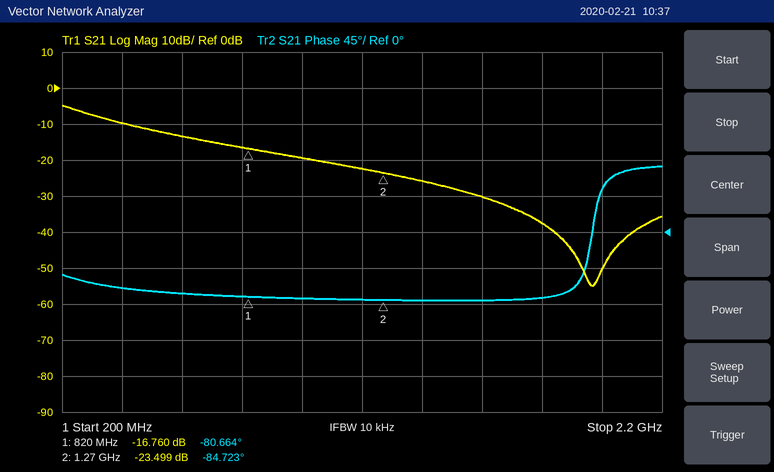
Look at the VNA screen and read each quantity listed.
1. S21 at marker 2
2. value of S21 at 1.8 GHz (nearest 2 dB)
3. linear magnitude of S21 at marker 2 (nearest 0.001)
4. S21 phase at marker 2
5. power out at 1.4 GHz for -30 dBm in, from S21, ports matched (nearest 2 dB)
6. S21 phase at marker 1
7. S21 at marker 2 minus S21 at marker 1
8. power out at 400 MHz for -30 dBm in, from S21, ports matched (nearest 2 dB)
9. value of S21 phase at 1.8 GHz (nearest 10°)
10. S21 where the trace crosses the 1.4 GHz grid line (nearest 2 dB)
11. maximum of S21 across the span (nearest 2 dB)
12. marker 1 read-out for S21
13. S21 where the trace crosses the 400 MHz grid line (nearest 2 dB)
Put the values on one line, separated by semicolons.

-23.499 dB; -38 dB; 0.067; -84.723°; -56 dBm; -80.664°; -6.739 dB; -40 dBm; -80°; -26 dB; -4 dB; -16.760 dB; -10 dB
